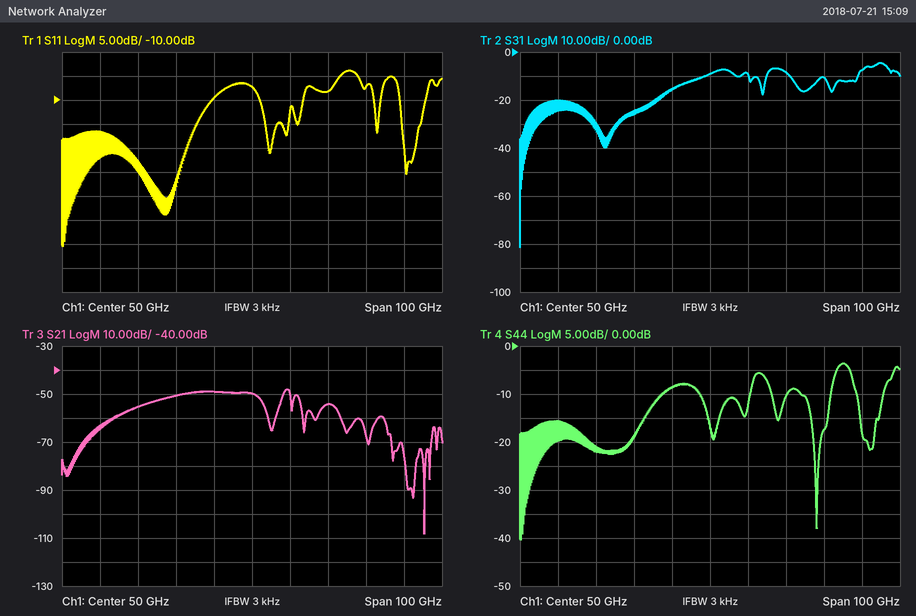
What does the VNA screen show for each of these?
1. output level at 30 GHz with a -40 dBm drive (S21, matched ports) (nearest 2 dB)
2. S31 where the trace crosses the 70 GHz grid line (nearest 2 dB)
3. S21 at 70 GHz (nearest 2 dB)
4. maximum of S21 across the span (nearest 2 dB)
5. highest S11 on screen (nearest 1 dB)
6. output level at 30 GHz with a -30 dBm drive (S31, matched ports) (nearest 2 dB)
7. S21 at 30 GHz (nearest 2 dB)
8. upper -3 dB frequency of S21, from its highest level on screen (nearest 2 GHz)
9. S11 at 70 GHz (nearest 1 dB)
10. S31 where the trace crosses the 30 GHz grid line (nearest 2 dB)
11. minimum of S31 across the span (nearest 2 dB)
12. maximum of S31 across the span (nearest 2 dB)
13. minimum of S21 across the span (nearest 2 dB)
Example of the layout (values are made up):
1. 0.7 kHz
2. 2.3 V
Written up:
1. -90 dBm
2. -8 dB
3. -54 dB
4. -48 dB
5. -4 dB
6. -56 dBm
7. -50 dB
8. 60 GHz
9. -8 dB
10. -26 dB
11. -82 dB
12. -4 dB
13. -108 dB
